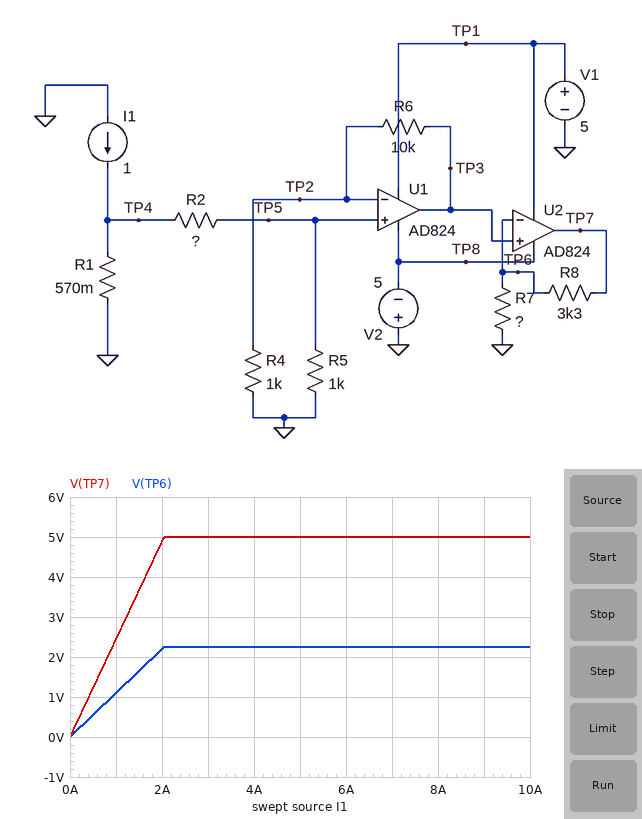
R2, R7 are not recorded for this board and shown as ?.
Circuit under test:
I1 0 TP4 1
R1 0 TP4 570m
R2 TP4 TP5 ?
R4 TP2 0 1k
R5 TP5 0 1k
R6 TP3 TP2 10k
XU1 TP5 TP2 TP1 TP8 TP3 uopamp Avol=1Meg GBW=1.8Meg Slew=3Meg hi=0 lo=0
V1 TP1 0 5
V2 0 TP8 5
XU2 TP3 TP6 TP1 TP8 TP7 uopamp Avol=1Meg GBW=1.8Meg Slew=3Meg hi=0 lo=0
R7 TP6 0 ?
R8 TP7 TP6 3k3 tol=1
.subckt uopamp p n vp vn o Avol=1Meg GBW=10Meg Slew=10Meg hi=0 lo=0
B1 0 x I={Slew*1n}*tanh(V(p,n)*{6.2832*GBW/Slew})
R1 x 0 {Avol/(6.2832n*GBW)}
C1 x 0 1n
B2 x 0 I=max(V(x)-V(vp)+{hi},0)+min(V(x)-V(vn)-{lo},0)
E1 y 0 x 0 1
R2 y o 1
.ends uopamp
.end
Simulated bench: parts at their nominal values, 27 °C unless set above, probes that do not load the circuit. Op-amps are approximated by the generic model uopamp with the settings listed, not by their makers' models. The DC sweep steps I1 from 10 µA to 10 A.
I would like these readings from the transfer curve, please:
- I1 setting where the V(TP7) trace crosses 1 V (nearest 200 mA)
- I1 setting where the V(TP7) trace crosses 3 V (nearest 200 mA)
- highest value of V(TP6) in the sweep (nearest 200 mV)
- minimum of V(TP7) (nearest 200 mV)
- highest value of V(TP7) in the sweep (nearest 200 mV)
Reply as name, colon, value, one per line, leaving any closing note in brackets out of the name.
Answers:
I1 setting where the V(TP7) trace crosses 1 V: 400 mA
I1 setting where the V(TP7) trace crosses 3 V: 1.2 A
highest value of V(TP6) in the sweep: 2.2 V
minimum of V(TP7): 0 V
highest value of V(TP7) in the sweep: 5.0 V
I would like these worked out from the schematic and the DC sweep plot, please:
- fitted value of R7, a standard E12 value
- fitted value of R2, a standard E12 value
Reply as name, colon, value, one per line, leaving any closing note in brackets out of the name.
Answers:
fitted value of R7, a standard E12 value: 2.7 kΩ
fitted value of R2, a standard E12 value: 4.7 kΩ
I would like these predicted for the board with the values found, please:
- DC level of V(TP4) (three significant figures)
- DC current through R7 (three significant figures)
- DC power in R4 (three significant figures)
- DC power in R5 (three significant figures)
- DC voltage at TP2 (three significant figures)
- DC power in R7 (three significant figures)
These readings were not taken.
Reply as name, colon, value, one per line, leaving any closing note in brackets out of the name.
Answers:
DC level of V(TP4): 570 mV
DC current through R7: 407 µA
DC power in R4: 10.0 µW
DC power in R5: 10.0 µW
DC voltage at TP2: 100 mV
DC power in R7: 448 µW
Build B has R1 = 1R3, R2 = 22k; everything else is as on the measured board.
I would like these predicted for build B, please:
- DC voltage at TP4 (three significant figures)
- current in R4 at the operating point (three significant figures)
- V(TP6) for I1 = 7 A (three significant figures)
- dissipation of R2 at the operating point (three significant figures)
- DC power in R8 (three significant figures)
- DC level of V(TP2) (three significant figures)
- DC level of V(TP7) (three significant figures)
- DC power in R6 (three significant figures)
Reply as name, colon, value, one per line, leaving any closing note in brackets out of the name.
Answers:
DC voltage at TP4: 1.30 V
current in R4 at the operating point: 56.5 µA
V(TP6) for I1 = 7 A: 2.25 V
dissipation of R2 at the operating point: 70.3 µW
DC power in R8: 175 µW
DC level of V(TP2): 56.5 mV
DC level of V(TP7): 1.38 V
DC power in R6: 31.9 µW
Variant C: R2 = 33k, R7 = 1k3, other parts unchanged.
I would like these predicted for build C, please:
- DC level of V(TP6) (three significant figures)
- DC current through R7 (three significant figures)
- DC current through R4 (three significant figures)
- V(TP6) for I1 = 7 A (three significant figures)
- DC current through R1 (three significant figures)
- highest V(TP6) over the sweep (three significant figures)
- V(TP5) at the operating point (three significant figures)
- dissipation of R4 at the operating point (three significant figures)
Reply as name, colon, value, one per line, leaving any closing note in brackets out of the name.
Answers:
DC level of V(TP6): 184 mV
DC current through R7: 142 µA
DC current through R4: 16.8 µA
V(TP6) for I1 = 7 A: 1.29 V
DC current through R1: 1.00 A
highest V(TP6) over the sweep: 1.41 V
V(TP5) at the operating point: 16.8 mV
dissipation of R4 at the operating point: 281 nW
